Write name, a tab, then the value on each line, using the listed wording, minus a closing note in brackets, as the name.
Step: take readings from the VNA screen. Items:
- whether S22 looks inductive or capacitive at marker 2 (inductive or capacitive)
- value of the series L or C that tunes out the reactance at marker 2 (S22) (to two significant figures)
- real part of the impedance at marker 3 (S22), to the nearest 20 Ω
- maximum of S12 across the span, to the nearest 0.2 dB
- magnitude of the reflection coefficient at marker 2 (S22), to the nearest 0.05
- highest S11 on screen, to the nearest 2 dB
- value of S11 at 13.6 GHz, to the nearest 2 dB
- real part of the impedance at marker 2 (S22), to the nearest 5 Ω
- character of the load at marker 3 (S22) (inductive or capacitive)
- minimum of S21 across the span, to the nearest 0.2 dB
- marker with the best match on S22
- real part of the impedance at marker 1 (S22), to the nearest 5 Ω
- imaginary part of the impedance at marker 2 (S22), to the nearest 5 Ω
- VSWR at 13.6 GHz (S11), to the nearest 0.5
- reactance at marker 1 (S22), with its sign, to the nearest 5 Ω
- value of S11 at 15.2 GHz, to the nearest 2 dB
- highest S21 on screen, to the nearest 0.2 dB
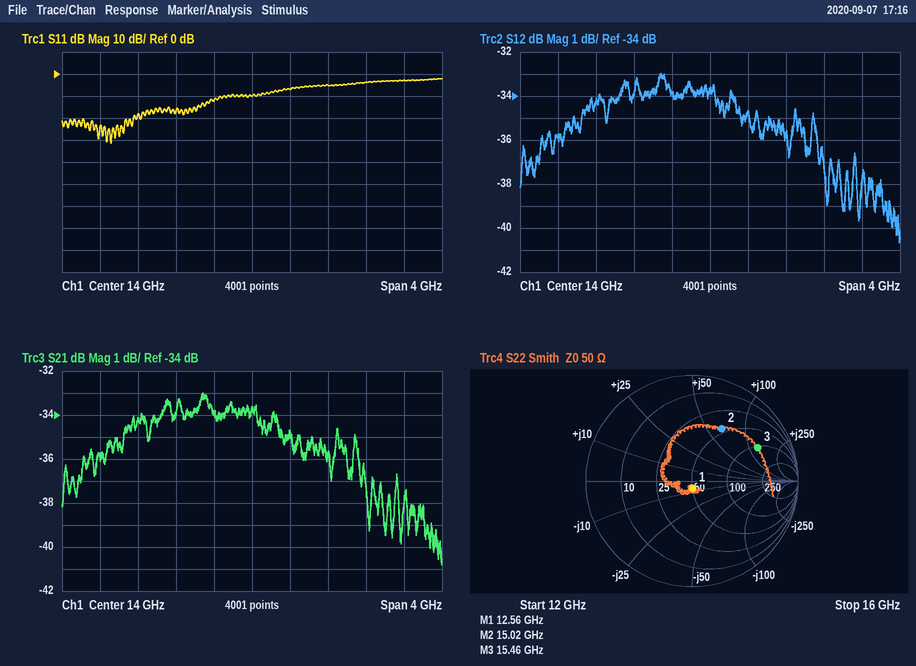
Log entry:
whether S22 looks inductive or capacitive at marker 2	inductive
value of the series L or C that tunes out the reactance at marker 2 (S22)	160 fF
real part of the impedance at marker 3 (S22), to the nearest 20 Ω	100 Ω
maximum of S12 across the span, to the nearest 0.2 dB	-33.0 dB
magnitude of the reflection coefficient at marker 2 (S22), to the nearest 0.05	0.55
highest S11 on screen, to the nearest 2 dB	-2 dB
value of S11 at 13.6 GHz, to the nearest 2 dB	-12 dB
real part of the impedance at marker 2 (S22), to the nearest 5 Ω	45 Ω
character of the load at marker 3 (S22)	inductive
minimum of S21 across the span, to the nearest 0.2 dB	-40.8 dB
marker with the best match on S22	marker 1
real part of the impedance at marker 1 (S22), to the nearest 5 Ω	50 Ω
imaginary part of the impedance at marker 2 (S22), to the nearest 5 Ω	+65 Ω
VSWR at 13.6 GHz (S11), to the nearest 0.5	1.5
reactance at marker 1 (S22), with its sign, to the nearest 5 Ω	-5 Ω
value of S11 at 15.2 GHz, to the nearest 2 dB	-4 dB
highest S21 on screen, to the nearest 0.2 dB	-33.0 dB
